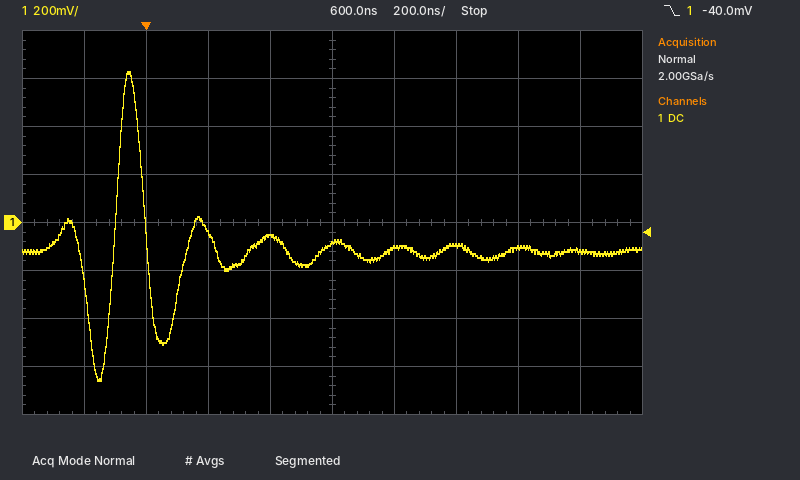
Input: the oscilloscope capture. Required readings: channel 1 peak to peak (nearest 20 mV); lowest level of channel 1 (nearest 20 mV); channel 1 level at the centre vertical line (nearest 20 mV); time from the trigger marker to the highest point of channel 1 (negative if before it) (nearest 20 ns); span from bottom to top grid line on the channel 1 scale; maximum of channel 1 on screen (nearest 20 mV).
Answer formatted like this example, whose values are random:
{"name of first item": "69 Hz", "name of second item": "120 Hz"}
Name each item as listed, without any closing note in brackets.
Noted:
{"channel 1 peak to peak": "1.28 V", "lowest level of channel 1": "-660 mV", "channel 1 level at the centre vertical line": "-80 mV", "time from the trigger marker to the highest point of channel 1 (negative if before it)": "-60 ns", "span from bottom to top grid line on the channel 1 scale": "1.6 V", "maximum of channel 1 on screen": "620 mV"}
